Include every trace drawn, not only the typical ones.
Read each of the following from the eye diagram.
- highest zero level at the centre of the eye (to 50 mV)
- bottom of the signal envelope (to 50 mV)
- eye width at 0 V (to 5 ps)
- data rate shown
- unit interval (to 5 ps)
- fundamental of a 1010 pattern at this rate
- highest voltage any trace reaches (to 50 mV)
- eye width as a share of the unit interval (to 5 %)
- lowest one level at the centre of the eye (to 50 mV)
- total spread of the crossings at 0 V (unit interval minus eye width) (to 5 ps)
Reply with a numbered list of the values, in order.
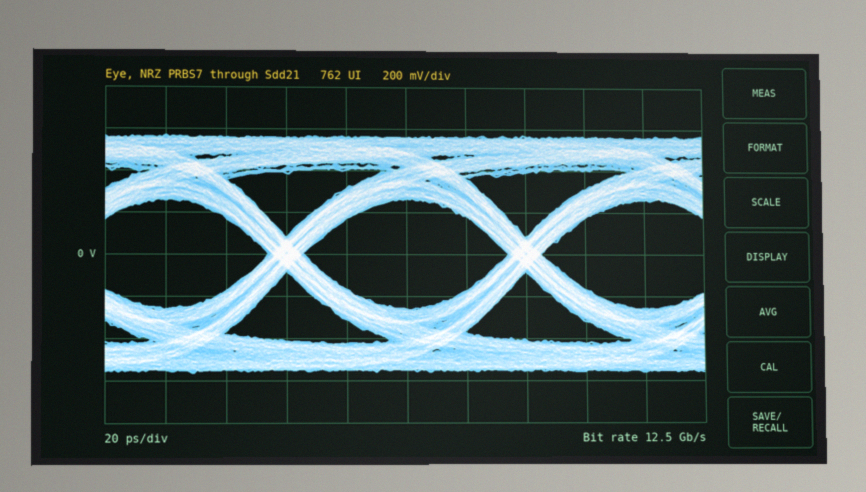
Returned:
1. -250 mV
2. -550 mV
3. 70 ps
4. 12.5 Gb/s
5. 80 ps
6. 6.25 GHz
7. 550 mV
8. 85 %
9. 250 mV
10. 10 ps
